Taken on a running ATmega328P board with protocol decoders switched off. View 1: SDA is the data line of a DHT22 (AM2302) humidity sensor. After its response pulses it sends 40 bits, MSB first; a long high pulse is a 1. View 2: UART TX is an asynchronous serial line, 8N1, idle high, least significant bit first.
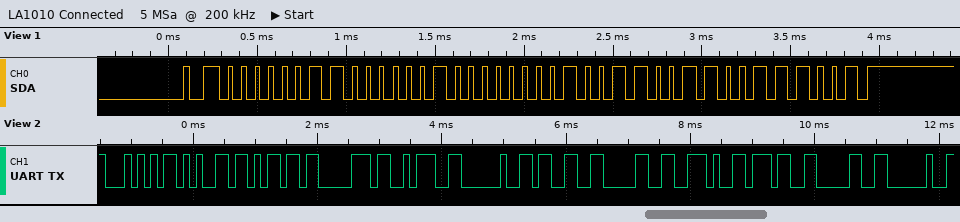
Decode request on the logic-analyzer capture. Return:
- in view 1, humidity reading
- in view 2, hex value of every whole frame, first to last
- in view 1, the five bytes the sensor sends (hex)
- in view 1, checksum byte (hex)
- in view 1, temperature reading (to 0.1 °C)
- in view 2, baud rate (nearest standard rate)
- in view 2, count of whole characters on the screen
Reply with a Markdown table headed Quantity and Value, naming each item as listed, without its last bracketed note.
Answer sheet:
| Quantity | Value |
|---|---|
| in view 1, humidity reading | 77.0 % |
| in view 2, hex value of every whole frame, first to last | 54 65 6D 70 3A 20 33 30 2E 37 30 20 |
| in view 1, the five bytes the sensor sends | 03 02 01 33 39 |
| in view 1, checksum byte | 0x39 |
| in view 1, temperature reading | 30.7 °C |
| in view 2, baud rate | 9600 baud |
| in view 2, count of whole characters on the screen | 12 |
